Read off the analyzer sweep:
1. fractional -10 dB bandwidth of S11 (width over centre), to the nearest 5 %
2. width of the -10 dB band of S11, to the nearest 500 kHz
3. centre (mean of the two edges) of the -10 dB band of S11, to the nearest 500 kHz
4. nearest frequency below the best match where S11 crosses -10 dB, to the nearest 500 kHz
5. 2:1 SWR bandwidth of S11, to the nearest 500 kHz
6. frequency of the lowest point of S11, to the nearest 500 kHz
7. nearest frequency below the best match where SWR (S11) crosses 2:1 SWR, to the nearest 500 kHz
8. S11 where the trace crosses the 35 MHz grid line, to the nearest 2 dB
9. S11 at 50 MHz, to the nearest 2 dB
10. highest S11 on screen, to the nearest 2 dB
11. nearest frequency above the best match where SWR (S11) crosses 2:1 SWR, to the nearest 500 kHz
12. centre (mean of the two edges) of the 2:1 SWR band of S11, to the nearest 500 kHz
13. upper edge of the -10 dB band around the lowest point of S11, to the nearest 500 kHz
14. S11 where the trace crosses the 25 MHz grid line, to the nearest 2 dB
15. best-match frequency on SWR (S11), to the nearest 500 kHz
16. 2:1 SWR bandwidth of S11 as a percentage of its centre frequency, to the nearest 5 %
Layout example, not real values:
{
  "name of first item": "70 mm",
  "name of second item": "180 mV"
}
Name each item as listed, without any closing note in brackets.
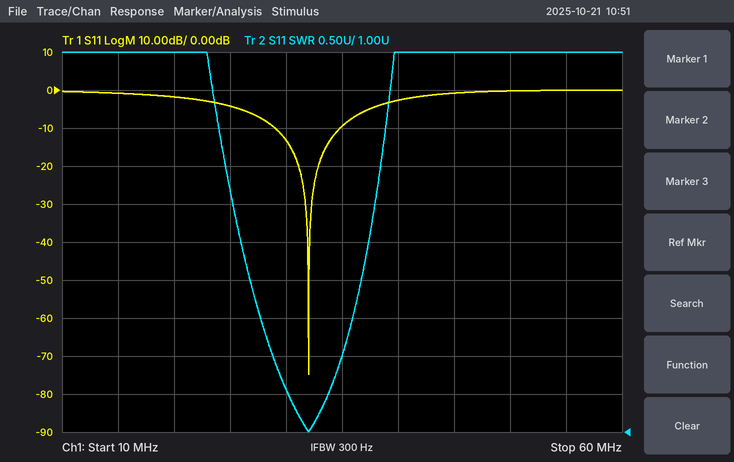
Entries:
{
  "fractional -10 dB bandwidth of S11 (width over centre), to the nearest 5 %": "20 %",
  "width of the -10 dB band of S11, to the nearest 500 kHz": "6.0 MHz",
  "centre (mean of the two edges) of the -10 dB band of S11, to the nearest 500 kHz": "32.0 MHz",
  "nearest frequency below the best match where S11 crosses -10 dB, to the nearest 500 kHz": "29.0 MHz",
  "2:1 SWR bandwidth of S11, to the nearest 500 kHz": "6.0 MHz",
  "frequency of the lowest point of S11, to the nearest 500 kHz": "32.0 MHz",
  "nearest frequency below the best match where SWR (S11) crosses 2:1 SWR, to the nearest 500 kHz": "29.0 MHz",
  "S11 where the trace crosses the 35 MHz grid line, to the nearest 2 dB": "-10 dB",
  "S11 at 50 MHz, to the nearest 2 dB": "0 dB",
  "highest S11 on screen, to the nearest 2 dB": "0 dB",
  "nearest frequency above the best match where SWR (S11) crosses 2:1 SWR, to the nearest 500 kHz": "35.0 MHz",
  "centre (mean of the two edges) of the 2:1 SWR band of S11, to the nearest 500 kHz": "32.0 MHz",
  "upper edge of the -10 dB band around the lowest point of S11, to the nearest 500 kHz": "35.0 MHz",
  "S11 where the trace crosses the 25 MHz grid line, to the nearest 2 dB": "-4 dB",
  "best-match frequency on SWR (S11), to the nearest 500 kHz": "32.0 MHz",
  "2:1 SWR bandwidth of S11 as a percentage of its centre frequency, to the nearest 5 %": "20 %"
}
